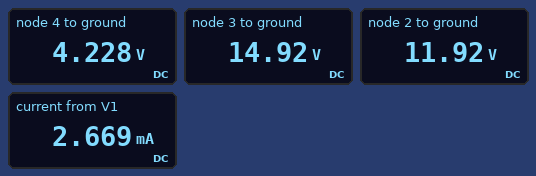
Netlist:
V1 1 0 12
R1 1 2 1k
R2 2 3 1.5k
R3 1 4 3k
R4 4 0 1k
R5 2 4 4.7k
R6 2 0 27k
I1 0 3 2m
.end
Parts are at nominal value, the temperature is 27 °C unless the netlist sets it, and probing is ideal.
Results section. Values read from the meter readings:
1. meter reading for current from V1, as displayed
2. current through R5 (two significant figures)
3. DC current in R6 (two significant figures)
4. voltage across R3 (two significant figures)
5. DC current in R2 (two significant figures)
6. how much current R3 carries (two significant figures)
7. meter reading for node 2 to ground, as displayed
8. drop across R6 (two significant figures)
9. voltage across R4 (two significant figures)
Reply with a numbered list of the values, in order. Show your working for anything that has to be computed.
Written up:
1. 2.669 mA
2. (11.92 V - 4.228 V) / 4.7 kΩ = 1.6 mA
3. (11.92 V) / 27 kΩ = 440 µA
4. 12 V - 4.228 V = 7.8 V
5. (14.92 V - 11.92 V) / 1.5 kΩ = 2.0 mA
6. (12 V - 4.228 V) / 3 kΩ = 2.6 mA
7. 11.92 V
8. 11.92 V = 12 V
9. 4.228 V = 4.2 V
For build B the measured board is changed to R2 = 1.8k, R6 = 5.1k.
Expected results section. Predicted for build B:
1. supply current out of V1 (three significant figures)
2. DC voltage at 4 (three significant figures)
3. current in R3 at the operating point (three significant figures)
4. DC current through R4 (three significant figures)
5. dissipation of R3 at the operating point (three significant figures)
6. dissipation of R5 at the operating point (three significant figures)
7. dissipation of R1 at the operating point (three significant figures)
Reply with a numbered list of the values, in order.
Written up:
1. 4.11 mA
2. 4.04 V
3. 2.65 mA
4. 4.04 mA
5. 21.1 mW
6. 9.01 mW
7. 2.11 mW
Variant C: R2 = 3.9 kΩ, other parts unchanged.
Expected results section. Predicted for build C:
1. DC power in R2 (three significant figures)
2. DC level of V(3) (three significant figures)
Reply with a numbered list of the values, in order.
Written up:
1. 15.6 mW
2. 19.7 V
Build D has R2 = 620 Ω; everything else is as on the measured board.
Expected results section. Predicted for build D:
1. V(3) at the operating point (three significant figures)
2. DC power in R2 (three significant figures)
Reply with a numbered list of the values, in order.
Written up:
1. 13.2 V
2. 2.48 mW
